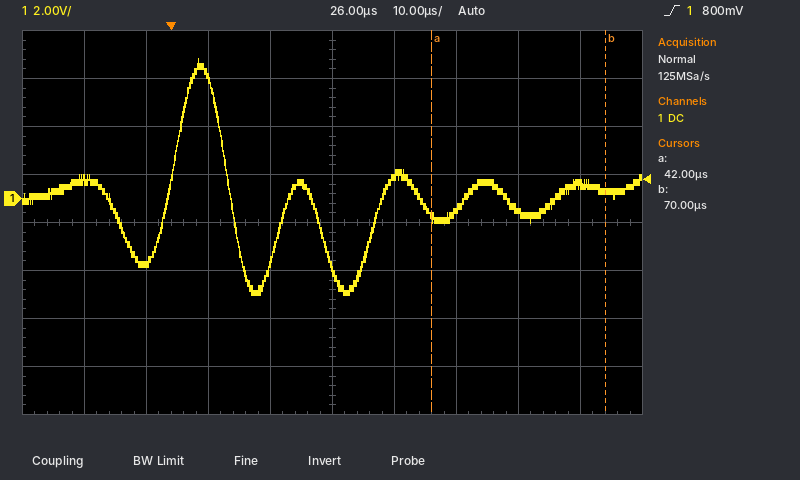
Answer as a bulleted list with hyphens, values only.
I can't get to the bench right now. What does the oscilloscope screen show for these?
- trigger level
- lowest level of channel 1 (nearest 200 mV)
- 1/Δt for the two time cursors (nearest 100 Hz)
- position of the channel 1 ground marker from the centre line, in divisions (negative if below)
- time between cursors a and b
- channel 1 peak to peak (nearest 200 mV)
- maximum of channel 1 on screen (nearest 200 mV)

- 800 mV
- -4.0 V
- 35.7 kHz
- +0.5 div
- 28 µs
- 9.8 V
- 5.8 V
